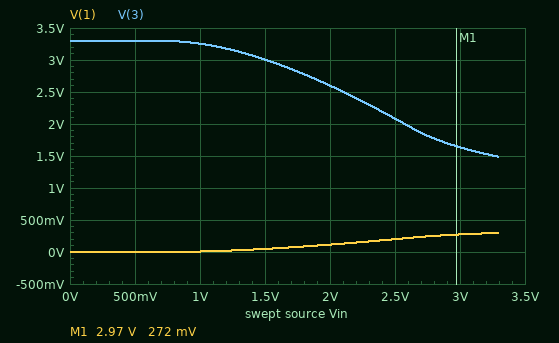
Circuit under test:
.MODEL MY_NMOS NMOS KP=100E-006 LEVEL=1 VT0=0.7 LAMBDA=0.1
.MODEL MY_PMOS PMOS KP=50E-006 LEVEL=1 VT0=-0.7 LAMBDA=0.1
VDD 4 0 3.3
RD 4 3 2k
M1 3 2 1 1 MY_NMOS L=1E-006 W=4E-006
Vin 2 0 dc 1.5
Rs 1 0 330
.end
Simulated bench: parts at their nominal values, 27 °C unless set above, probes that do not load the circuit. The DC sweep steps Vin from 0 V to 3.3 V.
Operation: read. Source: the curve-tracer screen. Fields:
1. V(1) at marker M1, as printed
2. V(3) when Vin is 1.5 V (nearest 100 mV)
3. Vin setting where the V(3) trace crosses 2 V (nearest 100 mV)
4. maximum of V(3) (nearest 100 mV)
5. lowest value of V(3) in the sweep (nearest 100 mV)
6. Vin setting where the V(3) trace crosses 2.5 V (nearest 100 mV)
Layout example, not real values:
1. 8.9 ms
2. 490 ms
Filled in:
1. 272 mV
2. 3.0 V
3. 2.6 V
4. 3.3 V
5. 1.5 V
6. 2.1 V
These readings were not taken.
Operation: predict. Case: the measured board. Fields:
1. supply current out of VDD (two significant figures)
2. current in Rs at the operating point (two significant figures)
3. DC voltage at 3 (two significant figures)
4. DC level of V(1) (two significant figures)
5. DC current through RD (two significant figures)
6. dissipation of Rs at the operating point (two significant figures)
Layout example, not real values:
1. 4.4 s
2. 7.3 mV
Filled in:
1. 150 µA
2. 150 µA
3. 3.0 V
4. 48 mV
5. 150 µA
6. 7.1 µW
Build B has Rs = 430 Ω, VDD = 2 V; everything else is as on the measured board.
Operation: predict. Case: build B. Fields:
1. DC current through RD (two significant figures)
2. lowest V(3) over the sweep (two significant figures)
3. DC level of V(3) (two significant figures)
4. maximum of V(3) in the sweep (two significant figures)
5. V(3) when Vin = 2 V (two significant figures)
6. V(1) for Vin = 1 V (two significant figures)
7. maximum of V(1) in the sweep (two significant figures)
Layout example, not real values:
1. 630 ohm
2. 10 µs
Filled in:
1. 130 µA
2. 880 mV
3. 1.7 V
4. 2.0 V
5. 1.4 V
6. 8.7 mV
7. 240 mV
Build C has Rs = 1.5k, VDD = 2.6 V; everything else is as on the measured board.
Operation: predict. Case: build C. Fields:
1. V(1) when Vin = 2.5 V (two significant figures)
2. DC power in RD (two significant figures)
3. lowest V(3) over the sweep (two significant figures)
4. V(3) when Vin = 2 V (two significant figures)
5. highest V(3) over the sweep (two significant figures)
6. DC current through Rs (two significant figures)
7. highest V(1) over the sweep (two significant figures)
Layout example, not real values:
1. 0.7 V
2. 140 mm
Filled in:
1. 540 mV
2. 21 µW
3. 1.6 V
4. 2.2 V
5. 2.6 V
6. 100 µA
7. 760 mV
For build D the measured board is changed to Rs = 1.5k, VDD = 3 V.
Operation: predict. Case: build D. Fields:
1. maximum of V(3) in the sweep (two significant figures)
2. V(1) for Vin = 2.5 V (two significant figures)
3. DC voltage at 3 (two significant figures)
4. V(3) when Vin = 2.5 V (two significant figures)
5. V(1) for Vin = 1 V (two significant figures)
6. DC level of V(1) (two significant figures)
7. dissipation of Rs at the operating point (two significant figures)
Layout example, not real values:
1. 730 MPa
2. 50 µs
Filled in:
1. 3.0 V
2. 550 mV
3. 2.8 V
4. 2.3 V
5. 29 mV
6. 160 mV
7. 16 µW
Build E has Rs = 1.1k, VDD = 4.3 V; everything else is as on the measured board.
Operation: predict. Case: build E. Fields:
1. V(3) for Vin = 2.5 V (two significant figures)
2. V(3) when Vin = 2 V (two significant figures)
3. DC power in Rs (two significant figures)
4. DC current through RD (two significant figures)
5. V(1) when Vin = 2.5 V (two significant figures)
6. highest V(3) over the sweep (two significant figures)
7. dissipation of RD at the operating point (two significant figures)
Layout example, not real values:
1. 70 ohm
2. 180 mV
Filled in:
1. 3.4 V
2. 3.8 V
3. 17 µW
4. 120 µA
5. 490 mV
6. 4.3 V
7. 30 µW
